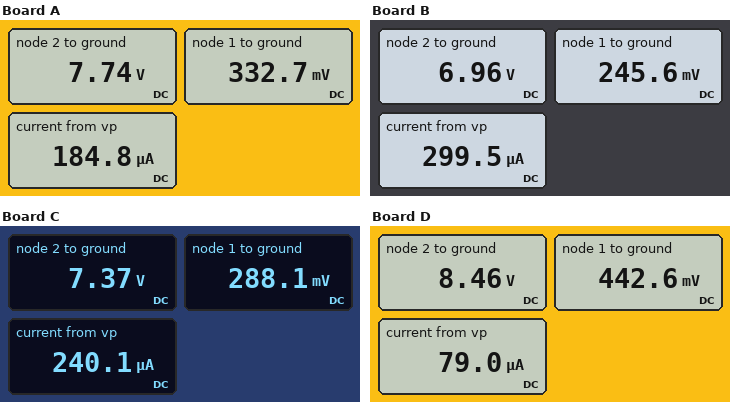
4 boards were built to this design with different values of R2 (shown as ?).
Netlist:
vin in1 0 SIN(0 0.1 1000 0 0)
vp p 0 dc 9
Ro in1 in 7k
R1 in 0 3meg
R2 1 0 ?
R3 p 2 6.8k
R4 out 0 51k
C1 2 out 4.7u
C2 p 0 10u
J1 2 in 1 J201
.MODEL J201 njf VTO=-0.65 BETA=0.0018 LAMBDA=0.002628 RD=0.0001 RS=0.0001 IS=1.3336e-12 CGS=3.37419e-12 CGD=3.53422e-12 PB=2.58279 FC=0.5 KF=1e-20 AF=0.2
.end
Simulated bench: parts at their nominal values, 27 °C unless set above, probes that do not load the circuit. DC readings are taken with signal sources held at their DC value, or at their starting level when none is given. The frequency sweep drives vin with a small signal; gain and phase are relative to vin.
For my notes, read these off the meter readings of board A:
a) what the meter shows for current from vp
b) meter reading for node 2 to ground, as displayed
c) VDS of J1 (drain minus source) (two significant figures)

184.8 µA
7.74 V
7.4 V
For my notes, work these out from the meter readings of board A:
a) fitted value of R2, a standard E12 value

1.8 kΩ
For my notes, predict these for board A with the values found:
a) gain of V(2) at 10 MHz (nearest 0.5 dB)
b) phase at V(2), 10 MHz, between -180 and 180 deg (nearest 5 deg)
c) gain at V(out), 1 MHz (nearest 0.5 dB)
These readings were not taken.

-4.0 dB
80 deg
6.5 dB
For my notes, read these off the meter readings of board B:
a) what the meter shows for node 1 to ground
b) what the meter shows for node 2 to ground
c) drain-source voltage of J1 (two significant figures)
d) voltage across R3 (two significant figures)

245.6 mV
6.96 V
6.7 V
2.0 V
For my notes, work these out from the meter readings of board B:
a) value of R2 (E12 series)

820 Ω
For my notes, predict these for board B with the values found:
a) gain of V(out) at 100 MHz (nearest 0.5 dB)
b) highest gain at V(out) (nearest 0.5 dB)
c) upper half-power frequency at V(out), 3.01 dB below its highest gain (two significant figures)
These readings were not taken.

-16.5 dB
12.0 dB
1.9 MHz
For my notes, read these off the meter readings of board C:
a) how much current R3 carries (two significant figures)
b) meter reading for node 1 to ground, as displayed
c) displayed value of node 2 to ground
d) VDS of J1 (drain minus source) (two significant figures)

240 µA
288.1 mV
7.37 V
7.1 V
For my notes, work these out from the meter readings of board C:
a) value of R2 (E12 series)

1.2 kΩ
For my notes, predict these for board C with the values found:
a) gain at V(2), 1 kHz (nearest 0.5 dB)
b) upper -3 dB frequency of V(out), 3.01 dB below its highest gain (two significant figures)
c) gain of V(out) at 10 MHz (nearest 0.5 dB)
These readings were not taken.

9.5 dB
2.3 MHz
-3.0 dB
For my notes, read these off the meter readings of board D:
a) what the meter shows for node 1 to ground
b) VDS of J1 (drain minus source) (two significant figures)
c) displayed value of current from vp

442.6 mV
8.0 V
79.0 µA
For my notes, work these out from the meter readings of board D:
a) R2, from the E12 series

5.6 kΩ
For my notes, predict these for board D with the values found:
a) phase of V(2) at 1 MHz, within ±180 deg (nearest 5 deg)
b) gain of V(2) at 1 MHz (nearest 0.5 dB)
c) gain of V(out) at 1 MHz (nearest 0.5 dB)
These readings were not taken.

160 deg
-1.5 dB
-1.5 dB
